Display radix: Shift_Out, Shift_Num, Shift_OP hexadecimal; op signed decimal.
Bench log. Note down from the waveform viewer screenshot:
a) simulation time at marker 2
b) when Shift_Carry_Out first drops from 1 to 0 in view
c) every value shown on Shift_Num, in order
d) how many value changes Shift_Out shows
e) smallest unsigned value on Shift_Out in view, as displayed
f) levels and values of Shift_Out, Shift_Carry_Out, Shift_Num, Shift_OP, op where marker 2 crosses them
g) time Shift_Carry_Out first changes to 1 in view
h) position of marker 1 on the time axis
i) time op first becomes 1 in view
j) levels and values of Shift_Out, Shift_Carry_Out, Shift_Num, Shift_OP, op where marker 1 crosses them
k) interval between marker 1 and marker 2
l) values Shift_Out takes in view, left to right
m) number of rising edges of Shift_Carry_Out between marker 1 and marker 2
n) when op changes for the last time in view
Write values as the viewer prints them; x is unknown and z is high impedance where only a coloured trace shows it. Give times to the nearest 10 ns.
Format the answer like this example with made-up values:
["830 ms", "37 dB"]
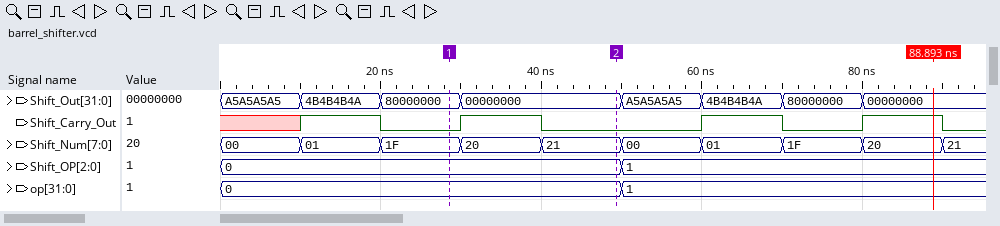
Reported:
["50 ns", "20 ns", "00, 01, 1F, 20, 21, 00, 01, 1F, 20, 21", "7", "00000000", "Shift_Out=00000000, Shift_Carry_Out=0, Shift_Num=21, Shift_OP=0, op=0", "10 ns", "30 ns", "50 ns", "Shift_Out=80000000, Shift_Carry_Out=0, Shift_Num=1F, Shift_OP=0, op=0", "20 ns", "A5A5A5A5, 4B4B4B4A, 80000000, 00000000, A5A5A5A5, 4B4B4B4A, 80000000, 00000000", "1", "50 ns"]
